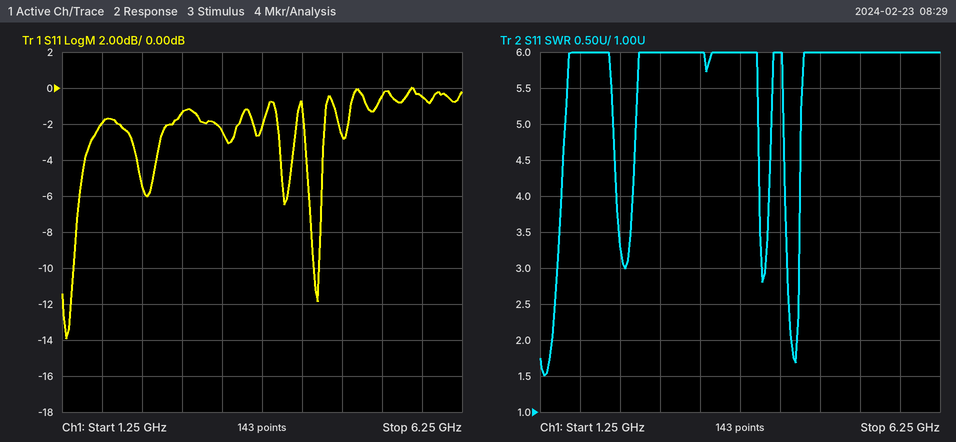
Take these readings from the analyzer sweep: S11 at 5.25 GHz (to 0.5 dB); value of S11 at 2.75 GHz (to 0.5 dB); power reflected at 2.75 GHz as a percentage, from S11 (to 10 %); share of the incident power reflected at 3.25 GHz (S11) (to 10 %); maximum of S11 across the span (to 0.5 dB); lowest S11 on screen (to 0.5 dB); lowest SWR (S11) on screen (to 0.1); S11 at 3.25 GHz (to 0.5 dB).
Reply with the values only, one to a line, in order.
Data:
-0.5 dB
-1.5 dB
70 %
60 %
0.0 dB
-14.0 dB
1.5
-2.5 dB
